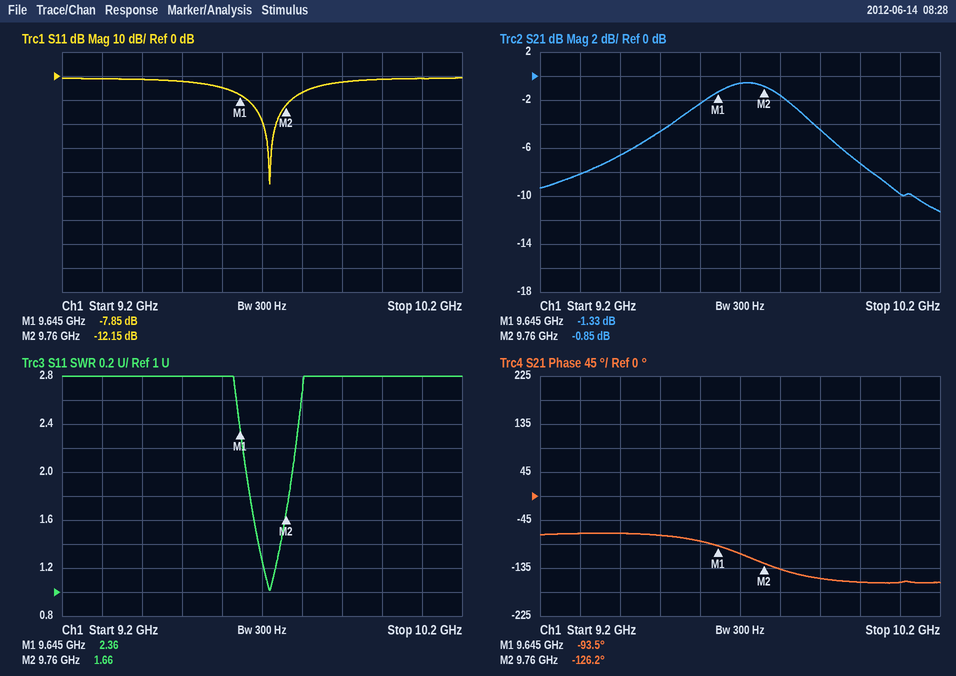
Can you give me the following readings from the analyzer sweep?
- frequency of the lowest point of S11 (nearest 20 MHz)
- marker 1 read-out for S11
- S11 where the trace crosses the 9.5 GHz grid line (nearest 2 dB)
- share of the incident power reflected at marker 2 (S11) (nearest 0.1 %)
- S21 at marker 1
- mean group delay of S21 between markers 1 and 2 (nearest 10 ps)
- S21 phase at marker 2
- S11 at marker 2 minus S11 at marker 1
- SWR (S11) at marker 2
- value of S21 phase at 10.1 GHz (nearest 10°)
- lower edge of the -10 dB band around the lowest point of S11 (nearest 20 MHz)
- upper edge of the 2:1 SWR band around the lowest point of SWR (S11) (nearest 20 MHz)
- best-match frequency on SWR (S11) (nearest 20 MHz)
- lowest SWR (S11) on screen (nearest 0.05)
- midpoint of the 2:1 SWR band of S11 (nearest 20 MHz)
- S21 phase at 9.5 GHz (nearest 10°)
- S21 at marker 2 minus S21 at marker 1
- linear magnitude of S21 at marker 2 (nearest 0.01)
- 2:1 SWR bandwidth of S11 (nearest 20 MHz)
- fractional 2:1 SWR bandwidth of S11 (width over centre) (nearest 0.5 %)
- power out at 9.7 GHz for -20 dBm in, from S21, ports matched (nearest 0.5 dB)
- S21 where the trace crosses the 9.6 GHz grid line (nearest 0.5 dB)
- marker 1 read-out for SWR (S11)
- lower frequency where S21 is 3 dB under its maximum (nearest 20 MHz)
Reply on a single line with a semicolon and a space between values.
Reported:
9.72 GHz; -7.85 dB; -2 dB; 6.1 %; -1.33 dB; 790 ps; -126.2°; -4.30 dB; 1.66; -160°; 9.66 GHz; 9.78 GHz; 9.72 GHz; 1.00; 9.72 GHz; -70°; 0.48 dB; 0.91; 120 MHz; 1.0 %; -20.5 dBm; -2.5 dB; 2.36; 9.54 GHz
